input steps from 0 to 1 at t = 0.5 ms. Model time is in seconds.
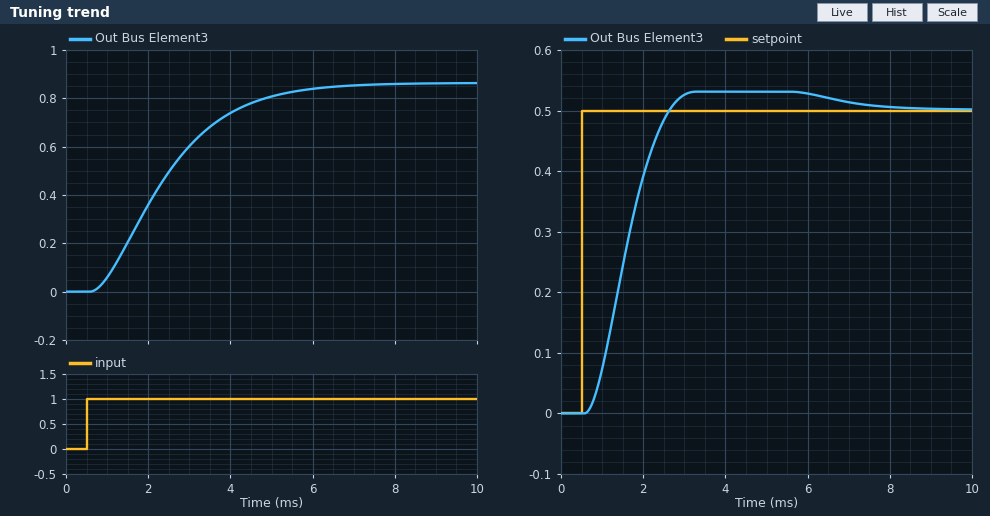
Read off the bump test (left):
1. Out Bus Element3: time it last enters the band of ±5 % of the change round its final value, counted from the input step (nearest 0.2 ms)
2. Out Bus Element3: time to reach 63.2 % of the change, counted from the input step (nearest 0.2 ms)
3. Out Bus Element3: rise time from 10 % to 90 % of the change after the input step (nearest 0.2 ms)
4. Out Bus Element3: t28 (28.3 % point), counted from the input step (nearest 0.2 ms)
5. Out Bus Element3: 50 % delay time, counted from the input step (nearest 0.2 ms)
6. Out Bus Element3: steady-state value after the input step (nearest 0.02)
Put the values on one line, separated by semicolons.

4.8 ms; 2.2 ms; 3.4 ms; 1.2 ms; 1.8 ms; 0.86
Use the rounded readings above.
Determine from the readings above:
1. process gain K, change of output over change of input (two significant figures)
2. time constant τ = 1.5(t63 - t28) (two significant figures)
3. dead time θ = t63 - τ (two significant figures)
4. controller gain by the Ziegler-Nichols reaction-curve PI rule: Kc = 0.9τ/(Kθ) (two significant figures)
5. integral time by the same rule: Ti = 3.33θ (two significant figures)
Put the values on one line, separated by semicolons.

0.86; 1.5 ms; 0.70 ms; 2.2; 2.3 ms
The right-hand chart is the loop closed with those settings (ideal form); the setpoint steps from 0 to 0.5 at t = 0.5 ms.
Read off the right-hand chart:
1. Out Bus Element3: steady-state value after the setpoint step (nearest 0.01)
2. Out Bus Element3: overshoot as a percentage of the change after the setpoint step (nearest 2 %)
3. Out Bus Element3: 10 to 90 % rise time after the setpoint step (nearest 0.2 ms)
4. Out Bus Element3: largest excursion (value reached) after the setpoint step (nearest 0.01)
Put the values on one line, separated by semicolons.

0.50; 6 %; 1.4 ms; 0.53
